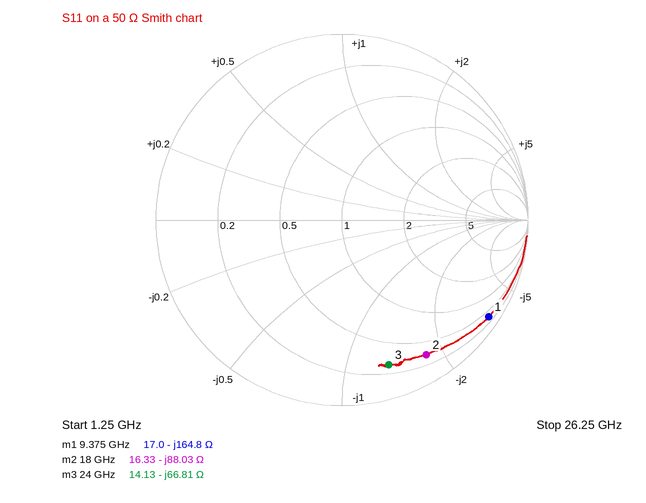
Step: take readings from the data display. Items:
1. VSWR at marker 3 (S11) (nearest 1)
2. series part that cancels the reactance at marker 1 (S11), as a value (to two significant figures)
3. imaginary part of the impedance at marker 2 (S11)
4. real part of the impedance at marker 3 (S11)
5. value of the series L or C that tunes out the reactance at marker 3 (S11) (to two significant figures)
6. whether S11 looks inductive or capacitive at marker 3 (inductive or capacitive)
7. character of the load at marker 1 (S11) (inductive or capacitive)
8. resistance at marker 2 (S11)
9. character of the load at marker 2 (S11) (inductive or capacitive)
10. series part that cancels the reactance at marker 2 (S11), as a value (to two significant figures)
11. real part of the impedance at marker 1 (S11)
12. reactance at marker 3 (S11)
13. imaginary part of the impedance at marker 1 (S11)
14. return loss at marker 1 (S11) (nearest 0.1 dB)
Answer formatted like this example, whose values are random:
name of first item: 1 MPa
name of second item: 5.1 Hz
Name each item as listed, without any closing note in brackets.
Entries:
VSWR at marker 3 (S11): 10
series part that cancels the reactance at marker 1 (S11), as a value: 2.8 nH
imaginary part of the impedance at marker 2: -88.03 Ω
real part of the impedance at marker 3: 14.13 Ω
value of the series L or C that tunes out the reactance at marker 3 (S11): 440 pH
whether S11 looks inductive or capacitive at marker 3: capacitive
character of the load at marker 1 (S11): capacitive
resistance at marker 2: 16.33 Ω
character of the load at marker 2 (S11): capacitive
series part that cancels the reactance at marker 2 (S11), as a value: 780 pH
real part of the impedance at marker 1: 17.0 Ω
reactance at marker 3: -66.81 Ω
imaginary part of the impedance at marker 1: -164.8 Ω
return loss at marker 1 (S11): 0.5 dB
